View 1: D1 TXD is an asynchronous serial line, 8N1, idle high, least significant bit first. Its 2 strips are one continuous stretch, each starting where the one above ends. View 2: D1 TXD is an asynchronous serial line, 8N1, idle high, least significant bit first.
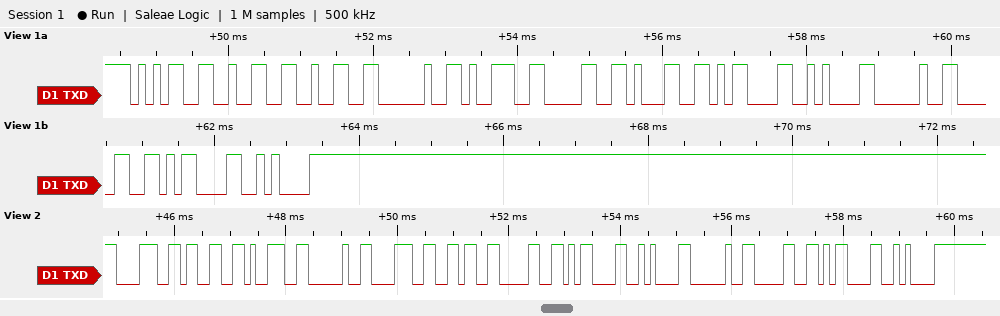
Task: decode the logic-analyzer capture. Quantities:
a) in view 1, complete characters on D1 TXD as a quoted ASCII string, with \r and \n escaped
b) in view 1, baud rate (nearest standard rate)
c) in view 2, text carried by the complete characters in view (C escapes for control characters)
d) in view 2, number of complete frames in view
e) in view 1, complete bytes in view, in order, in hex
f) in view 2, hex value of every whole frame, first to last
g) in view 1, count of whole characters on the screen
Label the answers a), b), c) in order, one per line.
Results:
a) "522 901\r\n 0\r\n"
b) 9600 baud
c) "839 860\r\n 0\r\n"
d) 13
e) 35 32 32 20 39 30 31 0D 0A 20 30 0D 0A
f) 0x38 0x33 0x39 0x20 0x38 0x36 0x30 0x0D 0x0A 0x20 0x30 0x0D 0x0A
g) 13
